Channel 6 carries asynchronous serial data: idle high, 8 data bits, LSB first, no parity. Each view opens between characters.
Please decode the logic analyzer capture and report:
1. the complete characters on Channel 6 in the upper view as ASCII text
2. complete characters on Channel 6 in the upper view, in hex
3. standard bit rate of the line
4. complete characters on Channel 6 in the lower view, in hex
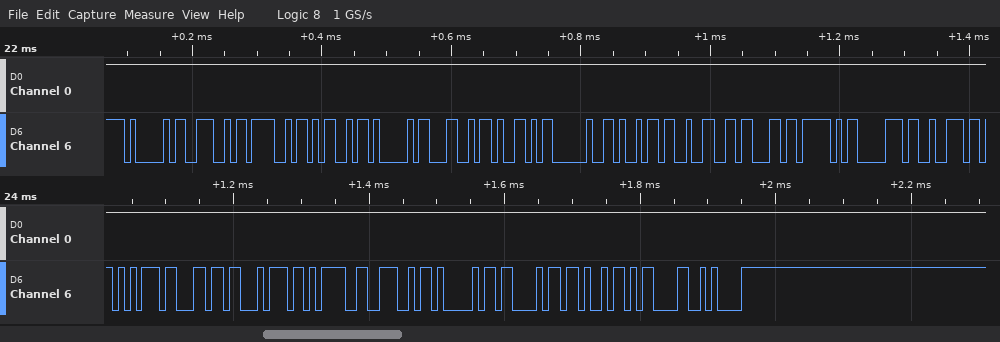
"ANOMALY i2c_pr"
41, 4E, 4F, 4D, 41, 4C, 59, 20, 69, 32, 63, 5F, 70, 72
115200 baud
75, 6C, 74, 3D, 4E, 41, 43, 4B, 0D, 0A
